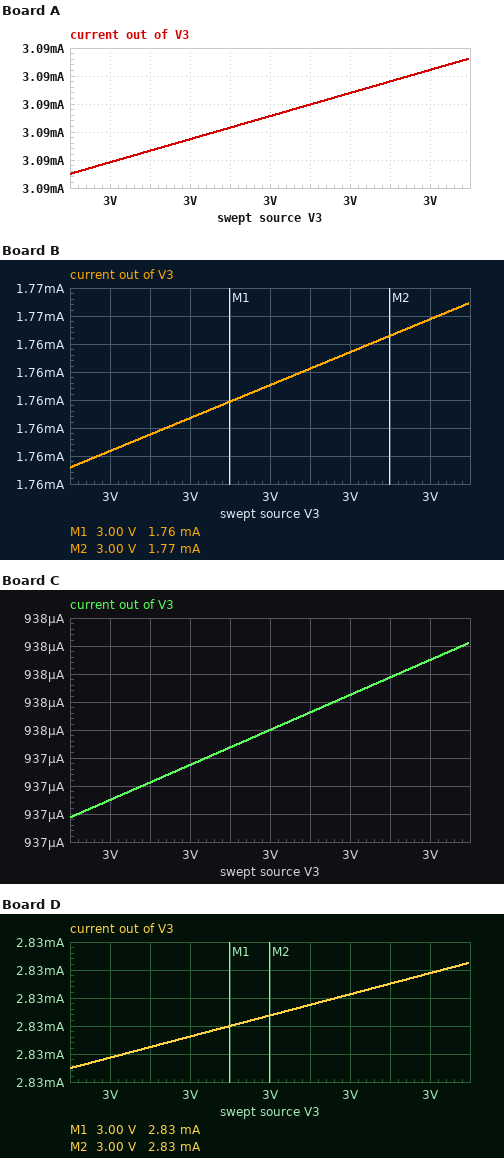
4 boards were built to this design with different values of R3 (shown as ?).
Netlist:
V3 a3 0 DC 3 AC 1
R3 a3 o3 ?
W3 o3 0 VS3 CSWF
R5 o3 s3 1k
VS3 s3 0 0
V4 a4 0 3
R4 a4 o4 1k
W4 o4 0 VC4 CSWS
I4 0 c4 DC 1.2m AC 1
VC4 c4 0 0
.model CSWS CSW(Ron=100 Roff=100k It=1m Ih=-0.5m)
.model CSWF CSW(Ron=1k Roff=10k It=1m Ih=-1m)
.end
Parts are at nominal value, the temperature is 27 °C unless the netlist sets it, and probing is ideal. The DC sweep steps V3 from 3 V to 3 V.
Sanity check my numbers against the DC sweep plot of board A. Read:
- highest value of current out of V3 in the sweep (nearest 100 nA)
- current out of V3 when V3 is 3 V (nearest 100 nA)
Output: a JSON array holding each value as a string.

["3.0938 mA", "3.0930 mA"]
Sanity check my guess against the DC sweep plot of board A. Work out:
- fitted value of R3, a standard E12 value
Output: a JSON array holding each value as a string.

["470 Ω"]
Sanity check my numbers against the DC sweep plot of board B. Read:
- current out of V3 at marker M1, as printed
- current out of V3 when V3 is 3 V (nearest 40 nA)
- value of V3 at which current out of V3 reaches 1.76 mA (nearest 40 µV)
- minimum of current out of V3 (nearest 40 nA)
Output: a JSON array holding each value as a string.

["1.76 mA", "1.76424 mA", "3.00016 V", "1.76412 mA"]
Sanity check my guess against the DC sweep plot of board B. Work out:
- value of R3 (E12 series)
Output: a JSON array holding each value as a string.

["1.2 kΩ"]
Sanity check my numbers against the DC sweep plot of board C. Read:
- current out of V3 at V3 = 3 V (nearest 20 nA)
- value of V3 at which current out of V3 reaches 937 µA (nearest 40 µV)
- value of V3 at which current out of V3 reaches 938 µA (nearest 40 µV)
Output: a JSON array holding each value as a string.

["937.50 µA", "2.99936 V", "3.00032 V"]
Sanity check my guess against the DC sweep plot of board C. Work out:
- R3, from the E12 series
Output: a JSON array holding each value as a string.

["2.7 kΩ"]
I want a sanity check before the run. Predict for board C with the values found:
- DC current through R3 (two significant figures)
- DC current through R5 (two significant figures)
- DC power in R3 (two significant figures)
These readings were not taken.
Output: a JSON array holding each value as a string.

["940 µA", "470 µA", "2.4 mW"]
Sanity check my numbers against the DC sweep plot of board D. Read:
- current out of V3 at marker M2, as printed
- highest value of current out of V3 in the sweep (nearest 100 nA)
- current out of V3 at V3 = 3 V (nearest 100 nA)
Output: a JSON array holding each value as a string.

["2.83 mA", "2.8311 mA", "2.8304 mA"]
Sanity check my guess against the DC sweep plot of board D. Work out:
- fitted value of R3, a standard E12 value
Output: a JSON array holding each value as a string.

["560 Ω"]
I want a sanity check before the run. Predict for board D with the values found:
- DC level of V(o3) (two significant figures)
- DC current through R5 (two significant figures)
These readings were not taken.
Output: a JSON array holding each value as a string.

["1.4 V", "1.4 mA"]
